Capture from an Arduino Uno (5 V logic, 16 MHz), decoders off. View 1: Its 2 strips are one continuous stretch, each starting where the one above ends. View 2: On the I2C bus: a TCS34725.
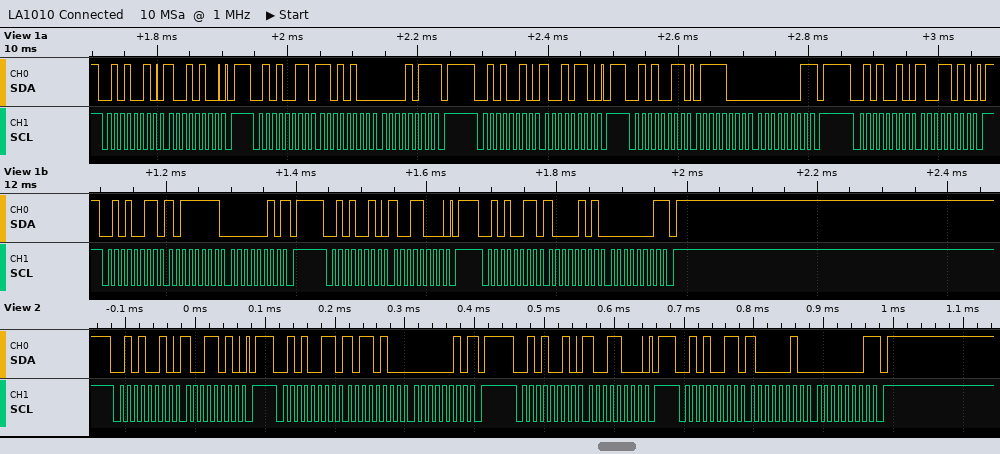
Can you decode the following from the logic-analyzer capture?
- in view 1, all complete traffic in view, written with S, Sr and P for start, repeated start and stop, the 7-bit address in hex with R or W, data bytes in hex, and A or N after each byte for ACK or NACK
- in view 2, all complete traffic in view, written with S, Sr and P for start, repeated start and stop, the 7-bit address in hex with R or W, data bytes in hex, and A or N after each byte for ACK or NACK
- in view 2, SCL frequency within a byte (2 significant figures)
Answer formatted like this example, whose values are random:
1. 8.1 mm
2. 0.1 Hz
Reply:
1. S 29W A 94 A P S 29R A D4 A 0B N P S 29W A 96 A P S 29R A 78 A 01 N P S 29W A 9A A P S 29R A BF A 02 N P S 29W A 98 A P S 29R A 85 A 01 N P
2. S 29W A 9A A P S 29R A B4 A 02 N P S 29W A 98 A P S 29R A 82 A 01 N P
3. 100 kHz
